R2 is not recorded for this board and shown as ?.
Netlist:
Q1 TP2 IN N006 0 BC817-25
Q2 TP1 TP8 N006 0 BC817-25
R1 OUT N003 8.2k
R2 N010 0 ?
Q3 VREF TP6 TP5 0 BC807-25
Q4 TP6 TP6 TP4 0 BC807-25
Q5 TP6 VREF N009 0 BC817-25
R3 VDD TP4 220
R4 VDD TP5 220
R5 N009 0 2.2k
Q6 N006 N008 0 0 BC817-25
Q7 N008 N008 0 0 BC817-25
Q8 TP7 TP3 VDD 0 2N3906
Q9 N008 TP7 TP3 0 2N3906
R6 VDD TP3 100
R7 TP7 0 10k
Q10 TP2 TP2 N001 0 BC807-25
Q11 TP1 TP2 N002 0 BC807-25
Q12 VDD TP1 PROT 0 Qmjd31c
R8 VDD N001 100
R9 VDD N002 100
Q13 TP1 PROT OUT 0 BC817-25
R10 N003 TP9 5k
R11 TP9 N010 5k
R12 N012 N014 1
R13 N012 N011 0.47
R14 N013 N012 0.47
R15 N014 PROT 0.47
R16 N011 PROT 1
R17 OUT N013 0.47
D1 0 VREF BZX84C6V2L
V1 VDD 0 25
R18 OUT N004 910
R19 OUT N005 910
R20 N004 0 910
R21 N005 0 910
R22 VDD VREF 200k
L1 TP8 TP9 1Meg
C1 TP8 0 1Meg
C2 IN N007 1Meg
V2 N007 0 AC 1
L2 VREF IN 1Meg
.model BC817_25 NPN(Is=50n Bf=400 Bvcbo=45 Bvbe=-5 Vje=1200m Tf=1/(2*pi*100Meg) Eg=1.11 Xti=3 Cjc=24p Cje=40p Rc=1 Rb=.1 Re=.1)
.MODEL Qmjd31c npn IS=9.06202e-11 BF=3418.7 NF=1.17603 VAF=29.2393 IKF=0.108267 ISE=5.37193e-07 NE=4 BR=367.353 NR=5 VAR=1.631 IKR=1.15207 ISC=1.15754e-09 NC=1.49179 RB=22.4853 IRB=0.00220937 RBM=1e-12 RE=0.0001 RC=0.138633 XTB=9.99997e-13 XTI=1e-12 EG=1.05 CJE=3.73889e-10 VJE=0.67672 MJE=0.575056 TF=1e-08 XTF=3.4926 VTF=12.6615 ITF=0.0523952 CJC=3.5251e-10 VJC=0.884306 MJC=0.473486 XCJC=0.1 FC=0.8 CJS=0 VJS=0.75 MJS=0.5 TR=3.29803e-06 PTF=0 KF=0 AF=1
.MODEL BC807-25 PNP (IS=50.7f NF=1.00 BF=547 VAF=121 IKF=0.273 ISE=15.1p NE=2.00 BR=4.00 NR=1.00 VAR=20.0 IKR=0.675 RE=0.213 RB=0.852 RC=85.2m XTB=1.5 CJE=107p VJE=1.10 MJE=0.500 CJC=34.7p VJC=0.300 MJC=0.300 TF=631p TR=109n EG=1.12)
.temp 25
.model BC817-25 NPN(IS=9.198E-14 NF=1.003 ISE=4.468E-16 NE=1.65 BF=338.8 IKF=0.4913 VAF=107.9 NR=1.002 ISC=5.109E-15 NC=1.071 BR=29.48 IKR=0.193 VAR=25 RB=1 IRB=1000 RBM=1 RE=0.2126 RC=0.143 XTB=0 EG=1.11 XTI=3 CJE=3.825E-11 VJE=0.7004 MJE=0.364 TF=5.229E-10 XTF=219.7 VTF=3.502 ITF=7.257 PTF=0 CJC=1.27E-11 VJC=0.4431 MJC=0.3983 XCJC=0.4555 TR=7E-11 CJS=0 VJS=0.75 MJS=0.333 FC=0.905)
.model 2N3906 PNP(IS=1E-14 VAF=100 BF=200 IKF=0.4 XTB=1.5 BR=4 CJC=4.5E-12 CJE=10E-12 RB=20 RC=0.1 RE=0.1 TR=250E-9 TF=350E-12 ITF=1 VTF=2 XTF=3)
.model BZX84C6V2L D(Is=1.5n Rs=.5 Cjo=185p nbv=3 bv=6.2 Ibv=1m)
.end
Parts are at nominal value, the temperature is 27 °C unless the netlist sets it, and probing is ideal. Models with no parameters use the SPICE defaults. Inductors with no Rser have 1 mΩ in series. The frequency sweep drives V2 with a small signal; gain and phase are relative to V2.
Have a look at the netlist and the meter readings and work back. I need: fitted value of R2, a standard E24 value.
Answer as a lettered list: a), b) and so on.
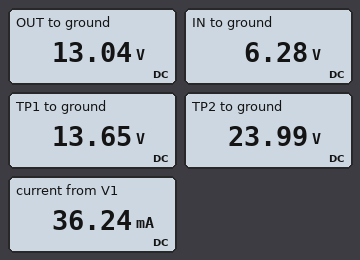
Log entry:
a) 7.5 kΩ
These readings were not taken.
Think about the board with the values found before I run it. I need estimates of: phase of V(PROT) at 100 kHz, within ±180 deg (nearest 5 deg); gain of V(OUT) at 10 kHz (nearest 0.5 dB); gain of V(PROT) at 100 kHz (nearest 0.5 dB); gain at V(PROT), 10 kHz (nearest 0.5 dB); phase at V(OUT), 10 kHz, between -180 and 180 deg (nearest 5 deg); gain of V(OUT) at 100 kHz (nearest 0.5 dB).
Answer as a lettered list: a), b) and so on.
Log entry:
a) -70 deg
b) 70.5 dB
c) 62.0 dB
d) 70.5 dB
e) -15 deg
f) 62.0 dB
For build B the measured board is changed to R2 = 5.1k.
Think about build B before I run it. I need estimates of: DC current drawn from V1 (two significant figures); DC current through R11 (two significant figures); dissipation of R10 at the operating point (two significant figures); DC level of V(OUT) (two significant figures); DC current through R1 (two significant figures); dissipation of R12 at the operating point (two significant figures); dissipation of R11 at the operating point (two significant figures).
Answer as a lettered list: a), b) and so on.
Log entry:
a) 38 mA
b) 620 µA
c) 2.0 mW
d) 15 V
e) 630 µA
f) 70 µW
g) 1.9 mW
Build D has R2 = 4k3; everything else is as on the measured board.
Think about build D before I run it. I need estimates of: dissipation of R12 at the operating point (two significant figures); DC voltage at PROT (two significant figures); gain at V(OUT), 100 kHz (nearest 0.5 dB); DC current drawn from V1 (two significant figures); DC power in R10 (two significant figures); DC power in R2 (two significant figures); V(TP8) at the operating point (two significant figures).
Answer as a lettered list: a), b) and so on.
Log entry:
a) 77 µW
b) 15 V
c) 61.5 dB
d) 39 mA
e) 2.3 mW
f) 2.0 mW
g) 6.3 V
